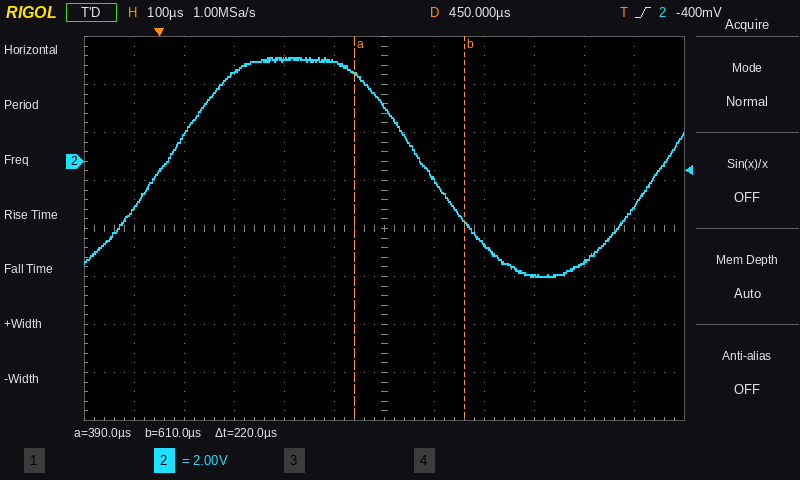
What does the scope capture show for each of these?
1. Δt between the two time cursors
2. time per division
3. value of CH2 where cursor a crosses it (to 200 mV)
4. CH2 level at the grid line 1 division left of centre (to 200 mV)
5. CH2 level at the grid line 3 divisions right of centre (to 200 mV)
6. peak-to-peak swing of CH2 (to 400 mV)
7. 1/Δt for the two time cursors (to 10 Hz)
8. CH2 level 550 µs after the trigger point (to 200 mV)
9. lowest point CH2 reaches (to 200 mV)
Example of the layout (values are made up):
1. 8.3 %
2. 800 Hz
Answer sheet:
1. 220 µs
2. 100 µs
3. 3.6 V
4. 4.2 V
5. -4.8 V
6. 9.2 V
7. 4.55 kHz
8. -800 mV
9. -4.8 V
